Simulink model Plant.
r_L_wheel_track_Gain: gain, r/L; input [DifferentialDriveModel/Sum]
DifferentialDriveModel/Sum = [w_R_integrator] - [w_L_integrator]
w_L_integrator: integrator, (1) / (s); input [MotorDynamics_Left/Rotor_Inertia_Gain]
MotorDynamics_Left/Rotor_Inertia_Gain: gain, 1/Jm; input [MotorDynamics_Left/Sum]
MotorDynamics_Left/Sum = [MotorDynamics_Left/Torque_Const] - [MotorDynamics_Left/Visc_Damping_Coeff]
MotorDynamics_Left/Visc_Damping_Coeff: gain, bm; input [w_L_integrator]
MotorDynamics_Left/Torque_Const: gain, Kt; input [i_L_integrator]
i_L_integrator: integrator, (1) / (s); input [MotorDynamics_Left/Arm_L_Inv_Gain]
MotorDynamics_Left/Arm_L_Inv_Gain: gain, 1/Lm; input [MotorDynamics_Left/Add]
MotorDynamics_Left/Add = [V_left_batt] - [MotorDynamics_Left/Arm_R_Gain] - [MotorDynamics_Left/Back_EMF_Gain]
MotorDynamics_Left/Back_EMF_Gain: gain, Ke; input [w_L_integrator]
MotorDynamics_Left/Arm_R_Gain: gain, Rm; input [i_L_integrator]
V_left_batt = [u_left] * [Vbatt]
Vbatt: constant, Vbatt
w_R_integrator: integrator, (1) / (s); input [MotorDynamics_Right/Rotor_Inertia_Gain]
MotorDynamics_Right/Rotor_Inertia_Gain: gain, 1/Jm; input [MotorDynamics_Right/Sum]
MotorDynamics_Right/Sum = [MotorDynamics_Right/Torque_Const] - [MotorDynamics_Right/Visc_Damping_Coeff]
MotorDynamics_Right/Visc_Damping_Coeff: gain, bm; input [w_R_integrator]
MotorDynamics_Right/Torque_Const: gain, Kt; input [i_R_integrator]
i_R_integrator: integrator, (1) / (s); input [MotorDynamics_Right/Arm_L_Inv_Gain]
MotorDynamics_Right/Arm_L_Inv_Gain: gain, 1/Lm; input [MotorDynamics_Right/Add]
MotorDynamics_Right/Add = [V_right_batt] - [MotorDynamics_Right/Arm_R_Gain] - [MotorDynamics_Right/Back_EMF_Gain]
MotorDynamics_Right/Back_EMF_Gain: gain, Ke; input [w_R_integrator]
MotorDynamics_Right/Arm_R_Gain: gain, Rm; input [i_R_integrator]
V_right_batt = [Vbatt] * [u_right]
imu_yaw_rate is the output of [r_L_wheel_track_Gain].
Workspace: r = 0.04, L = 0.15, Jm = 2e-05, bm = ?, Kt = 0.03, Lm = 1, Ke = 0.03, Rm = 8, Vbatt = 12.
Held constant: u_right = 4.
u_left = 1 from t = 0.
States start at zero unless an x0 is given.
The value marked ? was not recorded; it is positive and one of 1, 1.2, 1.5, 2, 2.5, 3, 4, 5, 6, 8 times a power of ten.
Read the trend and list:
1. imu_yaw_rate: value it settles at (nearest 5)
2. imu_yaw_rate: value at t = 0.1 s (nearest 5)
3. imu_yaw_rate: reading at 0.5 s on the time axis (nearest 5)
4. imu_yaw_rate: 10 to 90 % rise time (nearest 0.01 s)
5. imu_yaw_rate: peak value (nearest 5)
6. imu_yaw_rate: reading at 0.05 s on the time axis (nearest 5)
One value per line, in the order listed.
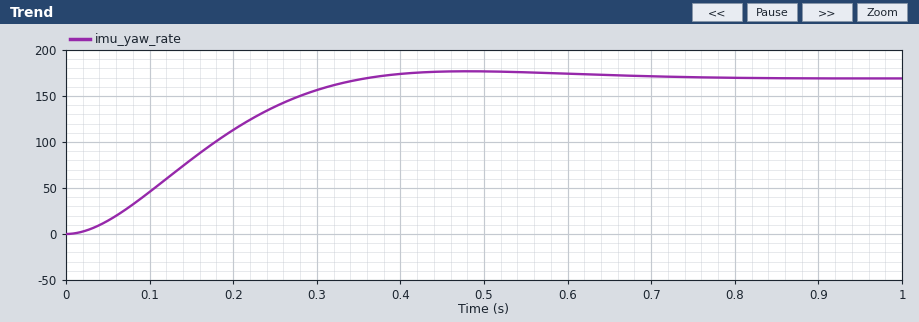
170
45
175
0.23 s
175
15
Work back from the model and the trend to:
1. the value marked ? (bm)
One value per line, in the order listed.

0.0001
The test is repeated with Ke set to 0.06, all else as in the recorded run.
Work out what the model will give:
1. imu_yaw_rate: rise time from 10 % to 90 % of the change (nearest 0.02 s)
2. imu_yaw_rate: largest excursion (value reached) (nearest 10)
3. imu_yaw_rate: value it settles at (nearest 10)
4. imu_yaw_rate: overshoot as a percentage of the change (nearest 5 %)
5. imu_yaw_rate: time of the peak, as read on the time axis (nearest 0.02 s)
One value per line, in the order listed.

0.16 s
120
110
10 %
0.34 s
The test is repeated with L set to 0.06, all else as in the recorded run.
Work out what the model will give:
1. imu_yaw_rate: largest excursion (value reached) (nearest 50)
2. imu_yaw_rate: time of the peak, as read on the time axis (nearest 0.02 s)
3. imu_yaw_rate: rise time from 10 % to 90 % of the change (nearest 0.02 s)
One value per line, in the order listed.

450
0.48 s
0.24 s
